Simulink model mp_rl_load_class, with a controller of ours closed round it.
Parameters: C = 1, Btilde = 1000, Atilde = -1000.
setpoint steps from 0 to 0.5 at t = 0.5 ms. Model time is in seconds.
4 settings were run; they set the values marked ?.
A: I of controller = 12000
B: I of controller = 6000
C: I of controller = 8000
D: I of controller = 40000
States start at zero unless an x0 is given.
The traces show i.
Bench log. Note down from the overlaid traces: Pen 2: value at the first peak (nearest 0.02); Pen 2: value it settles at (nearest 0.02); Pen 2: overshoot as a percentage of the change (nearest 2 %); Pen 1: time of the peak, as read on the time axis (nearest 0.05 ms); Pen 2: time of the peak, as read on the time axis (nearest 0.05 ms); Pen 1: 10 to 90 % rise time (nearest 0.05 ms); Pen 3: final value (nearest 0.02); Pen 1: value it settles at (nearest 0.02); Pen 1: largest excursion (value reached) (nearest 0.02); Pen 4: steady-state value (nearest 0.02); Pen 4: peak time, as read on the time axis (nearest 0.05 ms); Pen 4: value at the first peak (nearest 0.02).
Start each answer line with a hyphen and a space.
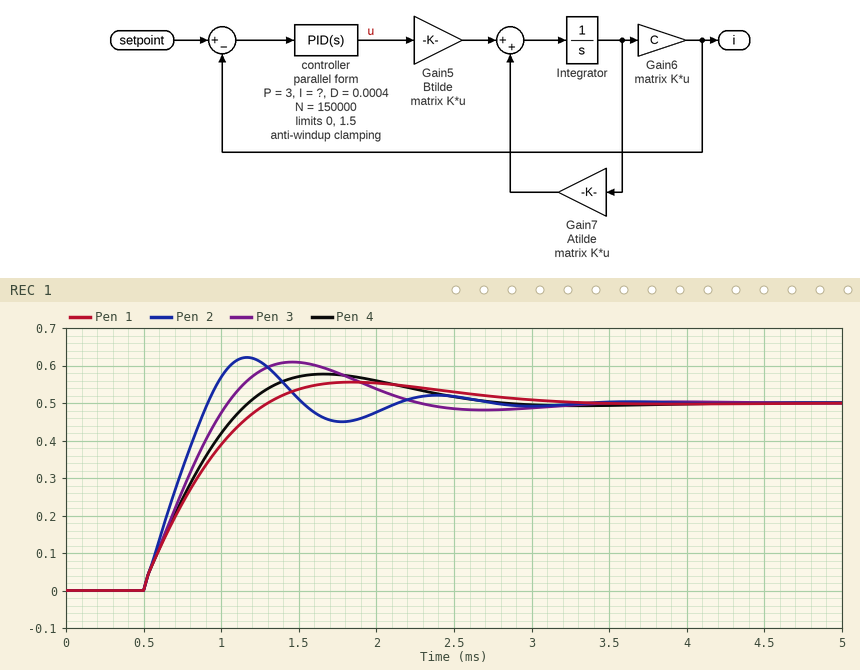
- 0.62
- 0.50
- 24 %
- 1.85 ms
- 1.15 ms
- 0.60 ms
- 0.50
- 0.50
- 0.56
- 0.50
- 1.65 ms
- 0.58
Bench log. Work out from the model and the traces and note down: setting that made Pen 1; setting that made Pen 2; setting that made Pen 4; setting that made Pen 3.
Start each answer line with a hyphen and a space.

- B
- D
- C
- A
